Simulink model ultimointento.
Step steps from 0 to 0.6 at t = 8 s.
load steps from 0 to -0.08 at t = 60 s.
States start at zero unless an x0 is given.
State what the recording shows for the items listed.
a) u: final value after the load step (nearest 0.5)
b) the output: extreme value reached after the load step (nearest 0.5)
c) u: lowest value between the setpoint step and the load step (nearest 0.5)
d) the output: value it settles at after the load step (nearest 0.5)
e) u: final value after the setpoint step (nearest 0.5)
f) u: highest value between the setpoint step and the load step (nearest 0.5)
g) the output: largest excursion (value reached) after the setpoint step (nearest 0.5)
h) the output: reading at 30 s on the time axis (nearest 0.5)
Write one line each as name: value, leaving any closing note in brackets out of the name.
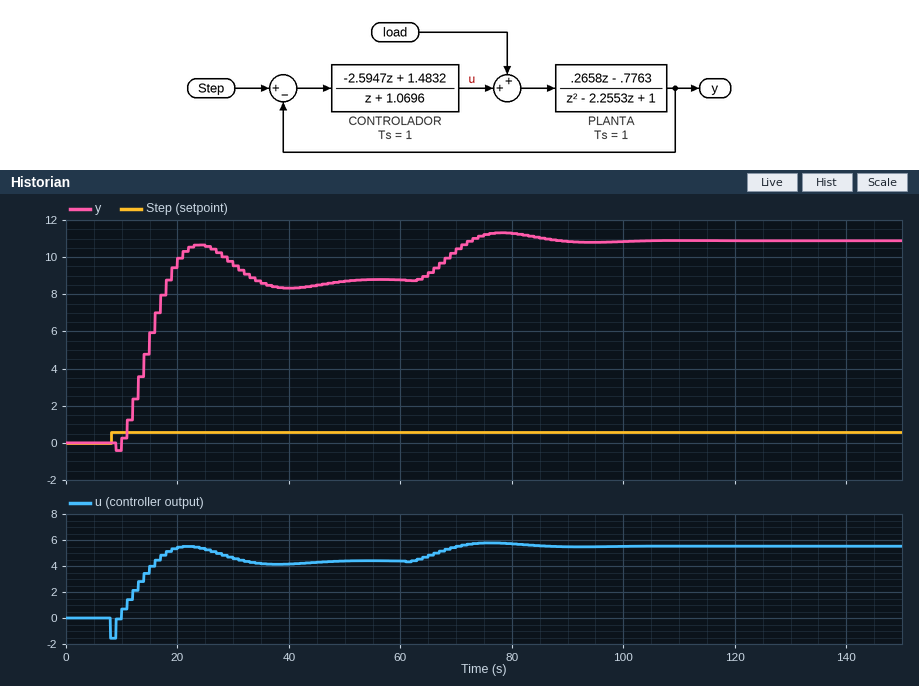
u: final value after the load step: 5.5
the output: extreme value reached after the load step: 11.5
u: lowest value between the setpoint step and the load step: -1.5
the output: value it settles at after the load step: 11.0
u: final value after the setpoint step: 4.5
u: highest value between the setpoint step and the load step: 5.5
the output: largest excursion (value reached) after the setpoint step: 10.5
the output: reading at 30 s on the time axis: 9.5
